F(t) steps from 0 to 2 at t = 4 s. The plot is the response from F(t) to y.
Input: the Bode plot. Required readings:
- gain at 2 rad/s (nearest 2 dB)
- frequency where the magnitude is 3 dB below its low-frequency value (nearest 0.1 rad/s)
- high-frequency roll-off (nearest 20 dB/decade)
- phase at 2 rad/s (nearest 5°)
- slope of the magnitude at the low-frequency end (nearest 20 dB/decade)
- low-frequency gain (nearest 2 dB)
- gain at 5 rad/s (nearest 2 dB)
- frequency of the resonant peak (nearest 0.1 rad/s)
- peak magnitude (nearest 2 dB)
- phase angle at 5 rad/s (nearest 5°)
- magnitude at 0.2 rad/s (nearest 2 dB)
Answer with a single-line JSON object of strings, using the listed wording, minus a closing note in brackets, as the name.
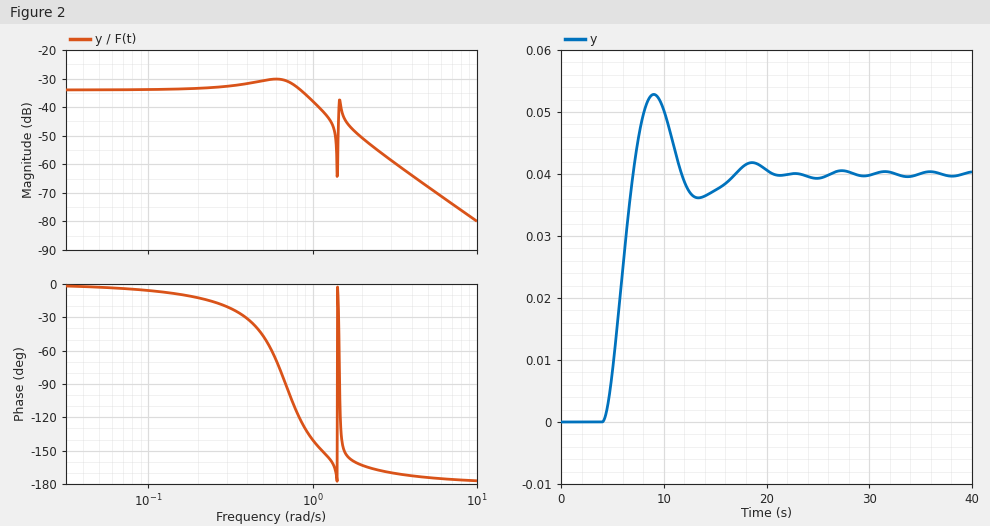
{"gain at 2 rad/s": "-50 dB", "frequency where the magnitude is 3 dB below its low-frequency value": "1.0 rad/s", "high-frequency roll-off": "-40 dB/decade", "phase at 2 rad/s": "-165°", "slope of the magnitude at the low-frequency end": "0 dB/decade", "low-frequency gain": "-34 dB", "gain at 5 rad/s": "-68 dB", "frequency of the resonant peak": "0.6 rad/s", "peak magnitude": "-30 dB", "phase angle at 5 rad/s": "-175°", "magnitude at 0.2 rad/s": "-34 dB"}
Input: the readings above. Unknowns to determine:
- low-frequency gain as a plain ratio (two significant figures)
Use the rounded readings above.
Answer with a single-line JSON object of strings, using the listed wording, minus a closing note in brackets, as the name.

{"low-frequency gain as a plain ratio": "0.020"}
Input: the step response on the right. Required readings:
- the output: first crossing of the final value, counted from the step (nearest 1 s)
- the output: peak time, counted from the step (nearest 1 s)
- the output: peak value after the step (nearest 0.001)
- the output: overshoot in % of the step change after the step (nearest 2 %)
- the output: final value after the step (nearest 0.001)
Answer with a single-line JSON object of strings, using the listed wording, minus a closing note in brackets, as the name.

{"the output: first crossing of the final value, counted from the step": "3 s", "the output: peak time, counted from the step": "5 s", "the output: peak value after the step": "0.053", "the output: overshoot in % of the step change after the step": "32 %", "the output: final value after the step": "0.040"}
